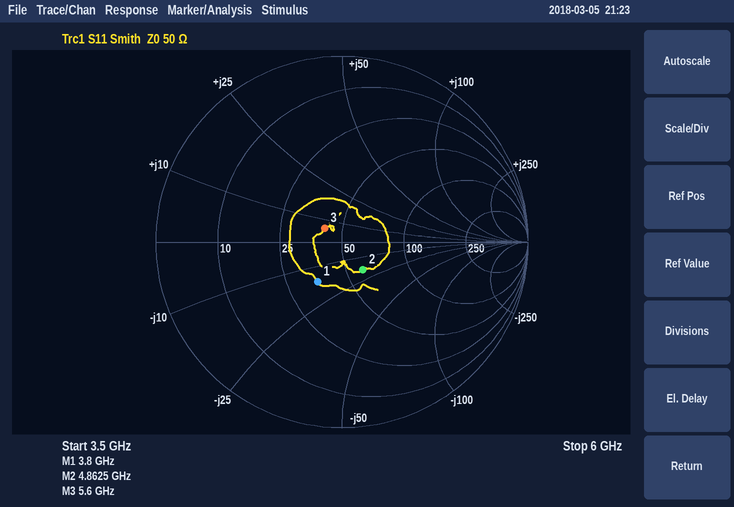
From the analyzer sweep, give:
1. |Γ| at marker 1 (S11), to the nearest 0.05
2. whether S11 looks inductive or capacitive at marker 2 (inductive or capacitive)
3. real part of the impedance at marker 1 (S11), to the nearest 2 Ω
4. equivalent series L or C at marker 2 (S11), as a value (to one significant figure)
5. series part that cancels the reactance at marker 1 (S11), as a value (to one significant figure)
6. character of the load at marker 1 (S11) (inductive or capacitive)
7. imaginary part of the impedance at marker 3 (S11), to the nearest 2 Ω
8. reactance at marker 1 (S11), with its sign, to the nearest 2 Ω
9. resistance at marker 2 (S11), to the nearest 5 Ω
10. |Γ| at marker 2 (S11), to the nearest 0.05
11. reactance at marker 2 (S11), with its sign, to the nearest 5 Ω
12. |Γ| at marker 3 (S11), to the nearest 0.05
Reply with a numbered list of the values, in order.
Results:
1. 0.25
2. capacitive
3. 36 Ω
4. 2 pF
5. 700 pH
6. capacitive
7. +6 Ω
8. -16 Ω
9. 60 Ω
10. 0.20
11. -20 Ω
12. 0.10
